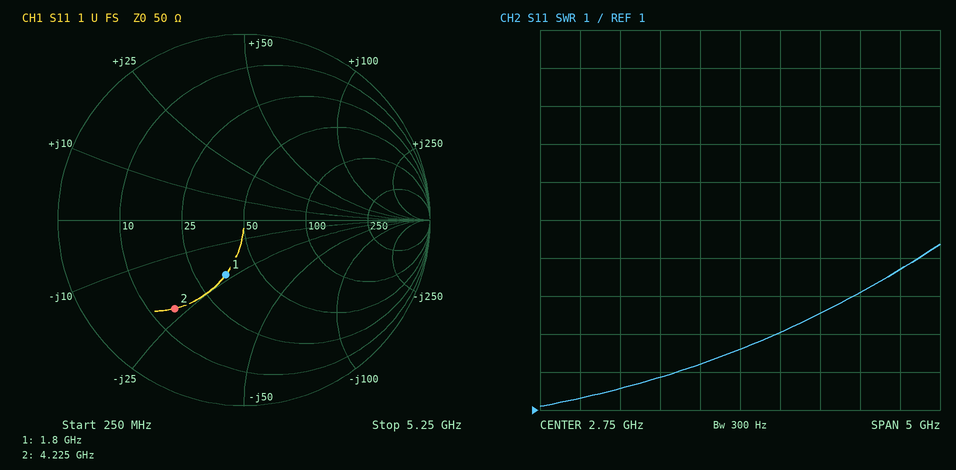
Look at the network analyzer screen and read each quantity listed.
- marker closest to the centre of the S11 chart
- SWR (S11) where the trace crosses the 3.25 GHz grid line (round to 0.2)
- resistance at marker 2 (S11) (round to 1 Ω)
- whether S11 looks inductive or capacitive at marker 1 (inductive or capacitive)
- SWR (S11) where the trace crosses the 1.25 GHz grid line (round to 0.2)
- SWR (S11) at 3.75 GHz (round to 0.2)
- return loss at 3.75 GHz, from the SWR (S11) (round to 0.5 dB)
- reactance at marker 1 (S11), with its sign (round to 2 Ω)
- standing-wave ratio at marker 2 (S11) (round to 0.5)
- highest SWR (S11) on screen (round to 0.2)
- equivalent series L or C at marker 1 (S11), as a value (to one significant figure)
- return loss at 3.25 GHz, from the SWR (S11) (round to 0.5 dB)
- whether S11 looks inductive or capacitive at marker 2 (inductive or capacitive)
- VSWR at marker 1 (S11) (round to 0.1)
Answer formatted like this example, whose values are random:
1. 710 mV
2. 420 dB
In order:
1. marker 1
2. 3.0
3. 15 Ω
4. capacitive
5. 1.6
6. 3.6
7. 5.0 dB
8. -22 Ω
9. 4.0
10. 5.4
11. 4 pF
12. 6.0 dB
13. capacitive
14. 1.9
